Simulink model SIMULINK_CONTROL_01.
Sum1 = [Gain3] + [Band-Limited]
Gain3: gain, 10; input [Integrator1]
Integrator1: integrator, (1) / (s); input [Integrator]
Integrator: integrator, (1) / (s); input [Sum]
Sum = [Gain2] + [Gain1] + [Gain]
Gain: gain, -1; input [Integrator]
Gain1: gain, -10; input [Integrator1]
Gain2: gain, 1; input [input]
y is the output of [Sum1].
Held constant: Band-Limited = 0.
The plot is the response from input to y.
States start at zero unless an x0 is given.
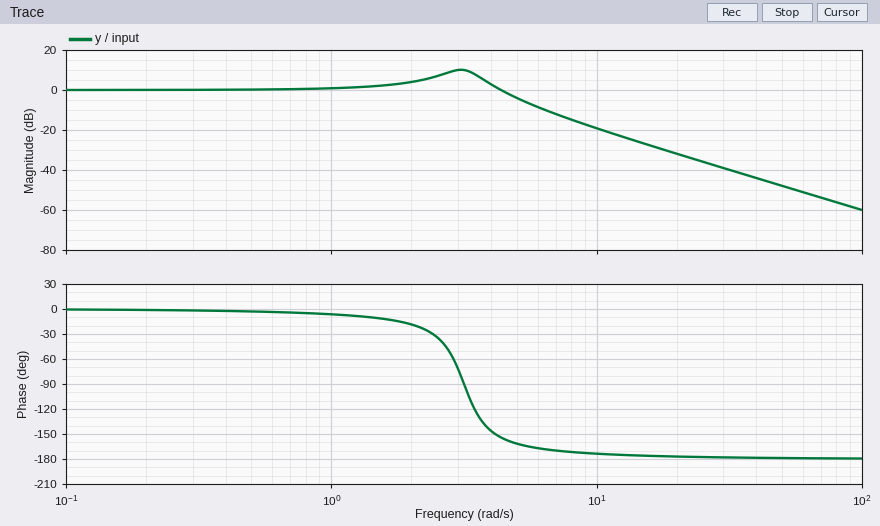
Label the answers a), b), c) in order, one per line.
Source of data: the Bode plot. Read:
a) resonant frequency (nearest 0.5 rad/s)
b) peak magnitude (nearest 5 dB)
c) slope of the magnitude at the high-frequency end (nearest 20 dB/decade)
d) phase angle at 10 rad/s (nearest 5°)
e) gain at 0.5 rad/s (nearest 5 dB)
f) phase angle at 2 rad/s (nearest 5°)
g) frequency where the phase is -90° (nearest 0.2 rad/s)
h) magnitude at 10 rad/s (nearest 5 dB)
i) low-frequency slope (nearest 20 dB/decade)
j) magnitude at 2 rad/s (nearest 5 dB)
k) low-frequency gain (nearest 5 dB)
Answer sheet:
a) 3.0 rad/s
b) 10 dB
c) -40 dB/decade
d) -175°
e) 0 dB
f) -20°
g) 3.2 rad/s
h) -20 dB
i) 0 dB/decade
j) 5 dB
k) 0 dB
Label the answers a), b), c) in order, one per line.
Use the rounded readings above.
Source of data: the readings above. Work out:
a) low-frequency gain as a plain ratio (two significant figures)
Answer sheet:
a) 1.0
